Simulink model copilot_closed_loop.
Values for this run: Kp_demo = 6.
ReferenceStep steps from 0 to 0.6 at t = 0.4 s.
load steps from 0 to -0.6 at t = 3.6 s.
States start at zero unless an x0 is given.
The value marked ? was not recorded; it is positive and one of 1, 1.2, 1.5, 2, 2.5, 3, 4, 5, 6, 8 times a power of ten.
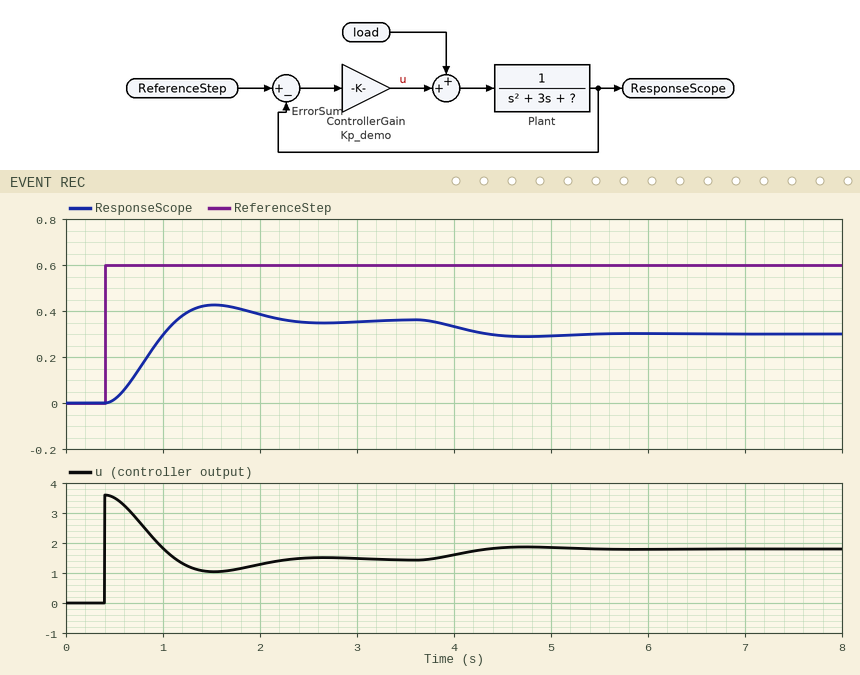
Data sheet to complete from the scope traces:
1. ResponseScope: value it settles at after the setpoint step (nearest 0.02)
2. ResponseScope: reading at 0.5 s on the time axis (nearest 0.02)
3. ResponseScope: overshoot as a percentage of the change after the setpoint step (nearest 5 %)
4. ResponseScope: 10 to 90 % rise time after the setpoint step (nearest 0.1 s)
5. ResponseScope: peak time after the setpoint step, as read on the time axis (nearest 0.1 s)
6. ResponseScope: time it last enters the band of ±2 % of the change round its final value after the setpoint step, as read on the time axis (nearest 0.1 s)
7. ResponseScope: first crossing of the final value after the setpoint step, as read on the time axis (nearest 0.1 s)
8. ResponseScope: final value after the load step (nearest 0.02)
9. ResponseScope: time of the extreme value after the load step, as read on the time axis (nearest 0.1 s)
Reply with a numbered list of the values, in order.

1. 0.36
2. 0.02
3. 20 %
4. 0.5 s
5. 1.5 s
6. 3.0 s
7. 1.1 s
8. 0.30
9. 4.7 s
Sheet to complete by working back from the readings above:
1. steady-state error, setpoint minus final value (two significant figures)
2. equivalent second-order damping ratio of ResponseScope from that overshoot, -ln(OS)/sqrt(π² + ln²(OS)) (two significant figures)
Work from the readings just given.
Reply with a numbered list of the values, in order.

1. 0.24
2. 0.46
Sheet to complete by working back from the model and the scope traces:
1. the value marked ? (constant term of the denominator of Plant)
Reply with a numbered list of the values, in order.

1. 4
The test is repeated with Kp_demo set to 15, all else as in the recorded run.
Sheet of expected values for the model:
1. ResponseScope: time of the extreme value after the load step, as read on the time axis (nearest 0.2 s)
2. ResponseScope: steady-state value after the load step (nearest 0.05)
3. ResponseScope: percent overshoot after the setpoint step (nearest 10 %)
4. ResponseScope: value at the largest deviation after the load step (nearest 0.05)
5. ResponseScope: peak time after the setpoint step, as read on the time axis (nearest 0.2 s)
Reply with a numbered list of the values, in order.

1. 4.4 s
2. 0.45
3. 30 %
4. 0.45
5. 1.2 s
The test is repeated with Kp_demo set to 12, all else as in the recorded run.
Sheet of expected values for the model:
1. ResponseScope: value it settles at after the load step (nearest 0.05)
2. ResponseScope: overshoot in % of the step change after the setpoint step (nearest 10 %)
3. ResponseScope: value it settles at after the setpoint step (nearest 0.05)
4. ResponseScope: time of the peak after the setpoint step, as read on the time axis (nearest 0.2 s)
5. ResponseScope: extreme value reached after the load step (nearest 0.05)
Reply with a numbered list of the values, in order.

1. 0.40
2. 30 %
3. 0.45
4. 1.2 s
5. 0.40
